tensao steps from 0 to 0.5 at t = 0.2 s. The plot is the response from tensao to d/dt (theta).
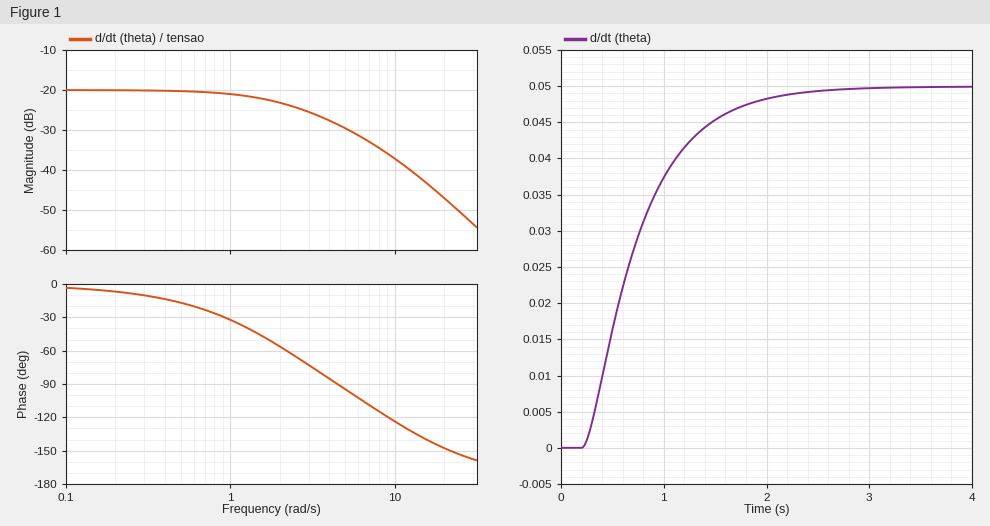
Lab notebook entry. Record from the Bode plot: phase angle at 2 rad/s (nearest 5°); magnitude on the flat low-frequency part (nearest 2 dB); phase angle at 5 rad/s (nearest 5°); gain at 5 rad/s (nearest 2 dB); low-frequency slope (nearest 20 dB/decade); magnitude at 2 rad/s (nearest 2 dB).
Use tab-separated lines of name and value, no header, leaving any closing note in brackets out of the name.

phase angle at 2 rad/s	-55°
magnitude on the flat low-frequency part	-20 dB
phase angle at 5 rad/s	-95°
gain at 5 rad/s	-30 dB
low-frequency slope	0 dB/decade
magnitude at 2 rad/s	-24 dB
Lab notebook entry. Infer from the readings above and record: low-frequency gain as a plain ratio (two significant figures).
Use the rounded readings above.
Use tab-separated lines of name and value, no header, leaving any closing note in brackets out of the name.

low-frequency gain as a plain ratio	0.10
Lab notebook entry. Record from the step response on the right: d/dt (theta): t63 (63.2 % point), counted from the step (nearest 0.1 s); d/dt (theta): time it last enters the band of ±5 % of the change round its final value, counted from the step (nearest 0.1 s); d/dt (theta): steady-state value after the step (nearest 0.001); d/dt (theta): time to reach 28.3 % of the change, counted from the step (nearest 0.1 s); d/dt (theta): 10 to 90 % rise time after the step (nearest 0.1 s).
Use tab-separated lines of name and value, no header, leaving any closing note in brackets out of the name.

d/dt (theta): t63 (63.2 % point), counted from the step	0.6 s
d/dt (theta): time it last enters the band of ±5 % of the change round its final value, counted from the step	1.6 s
d/dt (theta): steady-state value after the step	0.050
d/dt (theta): time to reach 28.3 % of the change, counted from the step	0.3 s
d/dt (theta): 10 to 90 % rise time after the step	1.1 s
